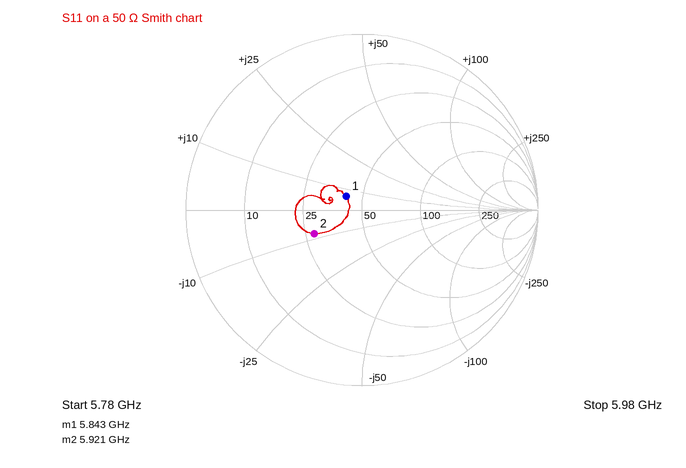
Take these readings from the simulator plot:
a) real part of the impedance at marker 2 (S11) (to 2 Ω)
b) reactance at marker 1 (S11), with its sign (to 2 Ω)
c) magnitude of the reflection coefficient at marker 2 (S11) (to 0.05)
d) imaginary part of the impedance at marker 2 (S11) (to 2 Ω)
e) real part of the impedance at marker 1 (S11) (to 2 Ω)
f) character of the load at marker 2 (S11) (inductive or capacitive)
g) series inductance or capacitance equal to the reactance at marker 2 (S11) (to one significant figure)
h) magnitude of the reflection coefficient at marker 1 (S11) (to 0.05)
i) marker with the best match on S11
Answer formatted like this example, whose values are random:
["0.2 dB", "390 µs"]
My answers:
["28 Ω", "+6 Ω", "0.30", "-8 Ω", "42 Ω", "capacitive", "3 pF", "0.10", "marker 1"]
